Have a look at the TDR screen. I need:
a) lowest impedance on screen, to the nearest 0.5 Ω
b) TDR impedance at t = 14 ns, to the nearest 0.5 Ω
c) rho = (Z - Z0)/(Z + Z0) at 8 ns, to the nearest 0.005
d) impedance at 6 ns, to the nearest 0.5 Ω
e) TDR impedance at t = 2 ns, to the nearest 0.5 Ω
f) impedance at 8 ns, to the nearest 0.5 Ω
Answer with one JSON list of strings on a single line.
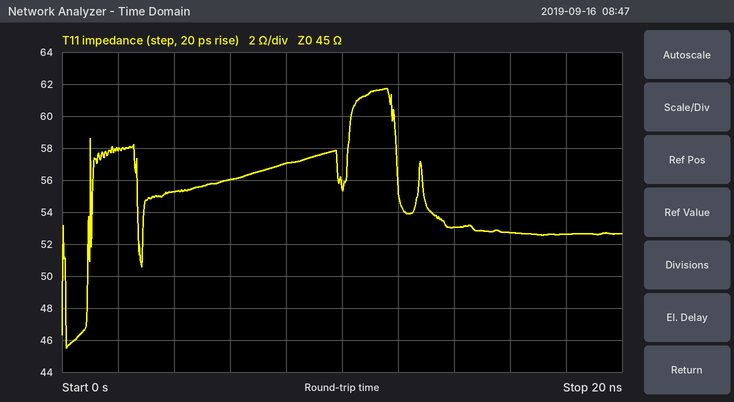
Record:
["45.5 Ω", "53.0 Ω", "+0.120", "56.0 Ω", "58.0 Ω", "57.0 Ω"]
